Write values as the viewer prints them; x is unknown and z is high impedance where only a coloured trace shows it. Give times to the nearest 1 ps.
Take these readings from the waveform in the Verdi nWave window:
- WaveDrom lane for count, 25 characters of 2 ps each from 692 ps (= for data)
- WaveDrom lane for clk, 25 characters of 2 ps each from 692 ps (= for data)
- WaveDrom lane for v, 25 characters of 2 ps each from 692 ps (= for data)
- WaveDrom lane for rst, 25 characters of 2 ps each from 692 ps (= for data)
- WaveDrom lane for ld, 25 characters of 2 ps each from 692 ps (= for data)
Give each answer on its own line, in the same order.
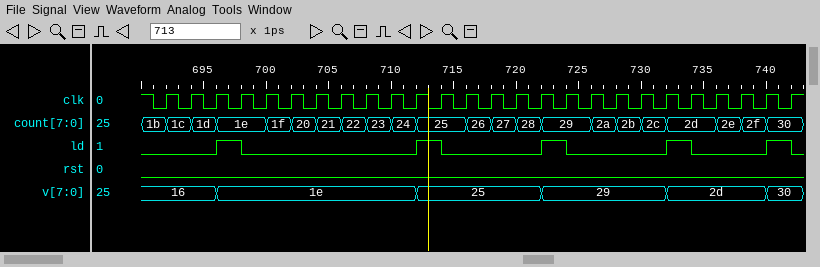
{name: 'count', wave: '===.=======.====.====.===', data: '1c 1d 1e 1f 20 21 22 23 24 25 26 27 28 29 2a 2b 2c 2d 2e 2f 30'}
{name: 'clk', wave: 'p........................'}
{name: 'v', wave: '=.=.......=....=....=...=', data: '16 1e 25 29 2d 30'}
{name: 'rst', wave: '0........................'}
{name: 'ld', wave: '0.10......10...10...10..1'}
